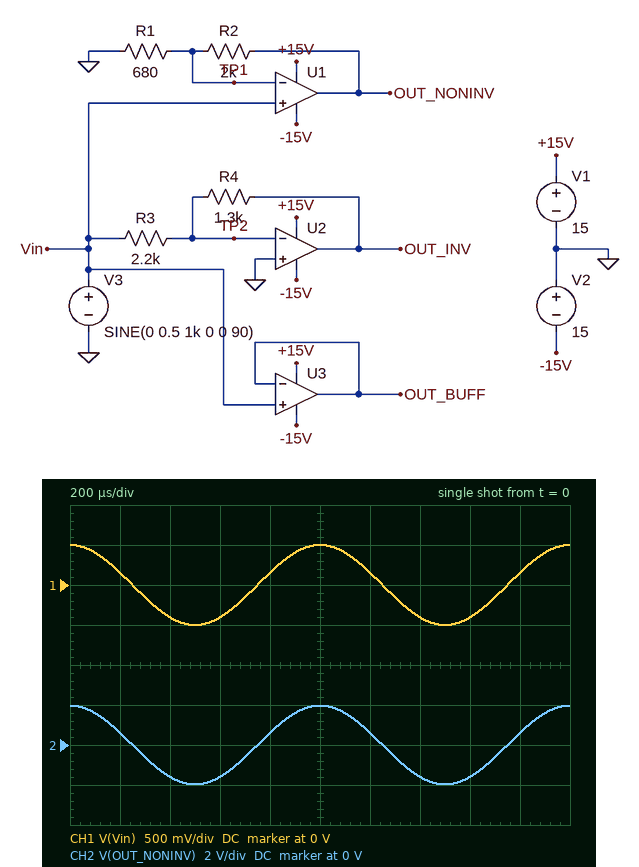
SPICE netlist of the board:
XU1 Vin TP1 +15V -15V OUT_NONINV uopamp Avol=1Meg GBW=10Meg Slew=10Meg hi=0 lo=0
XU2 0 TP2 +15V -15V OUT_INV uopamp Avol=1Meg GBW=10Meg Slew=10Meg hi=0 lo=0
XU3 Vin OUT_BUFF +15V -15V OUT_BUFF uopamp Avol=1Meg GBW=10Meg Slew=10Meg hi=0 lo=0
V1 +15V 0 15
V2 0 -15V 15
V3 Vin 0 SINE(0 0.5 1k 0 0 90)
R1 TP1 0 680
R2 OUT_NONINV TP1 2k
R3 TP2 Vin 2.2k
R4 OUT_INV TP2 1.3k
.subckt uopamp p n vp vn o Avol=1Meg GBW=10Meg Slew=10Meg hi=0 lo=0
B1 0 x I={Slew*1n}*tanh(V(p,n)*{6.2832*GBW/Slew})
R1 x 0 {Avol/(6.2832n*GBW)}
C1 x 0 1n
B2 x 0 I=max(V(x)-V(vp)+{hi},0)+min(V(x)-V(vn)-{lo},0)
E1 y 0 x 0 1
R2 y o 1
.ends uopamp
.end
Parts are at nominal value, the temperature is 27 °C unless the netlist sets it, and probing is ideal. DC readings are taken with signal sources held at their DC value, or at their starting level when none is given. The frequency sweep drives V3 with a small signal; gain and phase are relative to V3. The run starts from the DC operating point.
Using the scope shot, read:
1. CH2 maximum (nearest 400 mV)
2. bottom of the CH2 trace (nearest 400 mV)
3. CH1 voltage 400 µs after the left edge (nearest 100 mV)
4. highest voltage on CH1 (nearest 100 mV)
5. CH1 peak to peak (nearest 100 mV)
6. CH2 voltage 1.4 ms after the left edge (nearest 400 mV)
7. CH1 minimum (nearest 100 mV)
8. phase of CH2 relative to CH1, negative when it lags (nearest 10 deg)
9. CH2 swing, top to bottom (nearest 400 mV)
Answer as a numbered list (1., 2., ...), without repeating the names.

1. 2.0 V
2. -2.0 V
3. -400 mV
4. 500 mV
5. 1.0 V
6. -1.6 V
7. -500 mV
8. 0 deg
9. 4.0 V
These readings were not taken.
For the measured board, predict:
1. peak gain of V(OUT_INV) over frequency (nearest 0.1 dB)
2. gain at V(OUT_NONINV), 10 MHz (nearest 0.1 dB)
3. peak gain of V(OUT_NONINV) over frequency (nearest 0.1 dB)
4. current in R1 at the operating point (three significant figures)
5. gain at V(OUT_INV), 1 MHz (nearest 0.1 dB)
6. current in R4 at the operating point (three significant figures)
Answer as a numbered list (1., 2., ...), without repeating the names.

1. -4.6 dB
2. -0.3 dB
3. 11.9 dB
4. 735 µA
5. -4.7 dB
6. 227 µA
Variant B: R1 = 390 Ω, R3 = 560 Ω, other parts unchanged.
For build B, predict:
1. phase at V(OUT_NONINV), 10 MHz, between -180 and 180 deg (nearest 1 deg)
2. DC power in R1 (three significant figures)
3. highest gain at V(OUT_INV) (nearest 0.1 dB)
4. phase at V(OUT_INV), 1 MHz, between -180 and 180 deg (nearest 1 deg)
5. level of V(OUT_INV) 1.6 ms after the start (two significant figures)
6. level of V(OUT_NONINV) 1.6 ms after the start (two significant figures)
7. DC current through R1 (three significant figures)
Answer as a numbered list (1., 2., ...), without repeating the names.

1. -81 deg
2. 641 µW
3. 7.3 dB
4. 162 deg
5. 940 mV
6. -2.5 V
7. 1.28 mA
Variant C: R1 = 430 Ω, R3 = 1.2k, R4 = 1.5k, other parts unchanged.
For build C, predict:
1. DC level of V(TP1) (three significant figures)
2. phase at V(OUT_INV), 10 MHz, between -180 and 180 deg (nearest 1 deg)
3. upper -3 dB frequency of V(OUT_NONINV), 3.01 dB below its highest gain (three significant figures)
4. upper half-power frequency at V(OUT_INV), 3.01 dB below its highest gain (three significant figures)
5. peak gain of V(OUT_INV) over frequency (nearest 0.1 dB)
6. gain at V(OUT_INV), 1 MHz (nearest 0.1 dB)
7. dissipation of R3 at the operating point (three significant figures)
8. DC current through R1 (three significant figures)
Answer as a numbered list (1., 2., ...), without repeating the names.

1. 500 mV
2. 114 deg
3. 1.77 MHz
4. 4.44 MHz
5. 1.9 dB
6. 1.7 dB
7. 208 µW
8. 1.16 mA
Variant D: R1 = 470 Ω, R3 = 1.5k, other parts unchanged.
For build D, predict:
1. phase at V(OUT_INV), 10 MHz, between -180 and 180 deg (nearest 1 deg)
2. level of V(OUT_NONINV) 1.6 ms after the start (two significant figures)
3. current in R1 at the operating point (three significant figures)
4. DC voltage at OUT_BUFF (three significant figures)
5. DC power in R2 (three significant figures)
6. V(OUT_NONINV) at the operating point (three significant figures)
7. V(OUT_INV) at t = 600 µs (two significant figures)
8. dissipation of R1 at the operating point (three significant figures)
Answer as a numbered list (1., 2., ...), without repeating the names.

1. 118 deg
2. -2.1 V
3. 1.06 mA
4. 500 mV
5. 2.26 mW
6. 2.63 V
7. 350 mV
8. 532 µW
